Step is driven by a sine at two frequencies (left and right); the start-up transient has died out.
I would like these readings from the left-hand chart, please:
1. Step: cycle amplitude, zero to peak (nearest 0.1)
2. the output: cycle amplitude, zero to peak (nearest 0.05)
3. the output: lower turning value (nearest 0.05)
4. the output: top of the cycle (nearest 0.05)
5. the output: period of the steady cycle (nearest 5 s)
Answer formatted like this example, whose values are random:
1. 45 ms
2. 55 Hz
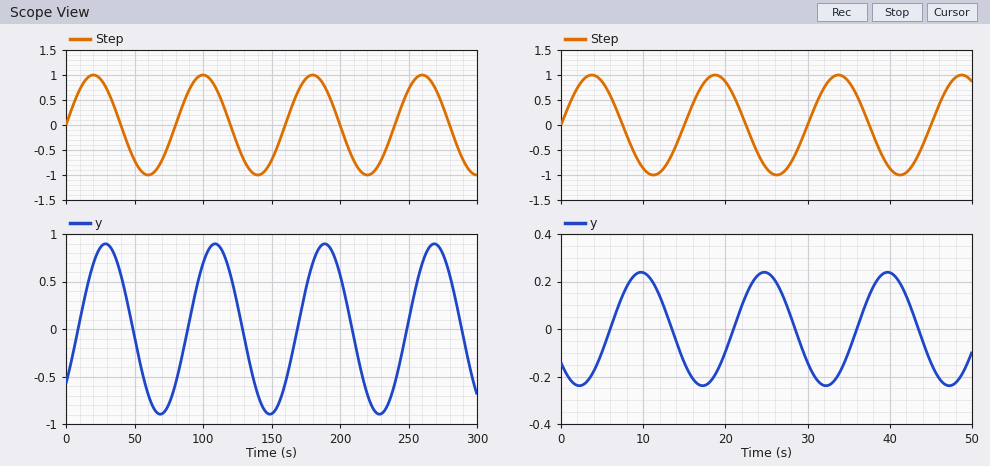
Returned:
1. 1.0
2. 0.90
3. -0.90
4. 0.90
5. 80 s
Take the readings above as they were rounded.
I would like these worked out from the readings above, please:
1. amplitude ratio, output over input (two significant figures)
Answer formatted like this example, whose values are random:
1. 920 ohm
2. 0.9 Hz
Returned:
1. 0.90
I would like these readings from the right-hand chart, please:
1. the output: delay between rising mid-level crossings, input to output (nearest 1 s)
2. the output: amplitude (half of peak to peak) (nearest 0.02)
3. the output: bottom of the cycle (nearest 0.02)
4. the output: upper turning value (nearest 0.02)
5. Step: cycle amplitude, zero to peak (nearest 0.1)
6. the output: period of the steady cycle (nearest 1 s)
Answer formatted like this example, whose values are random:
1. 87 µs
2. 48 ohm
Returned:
1. 6 s
2. 0.24
3. -0.24
4. 0.24
5. 1.0
6. 15 s
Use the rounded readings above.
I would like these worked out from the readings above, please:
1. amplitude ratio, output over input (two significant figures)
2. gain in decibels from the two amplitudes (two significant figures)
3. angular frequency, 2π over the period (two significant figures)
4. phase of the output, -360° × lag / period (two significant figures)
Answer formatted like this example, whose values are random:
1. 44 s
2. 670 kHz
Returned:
1. 0.24
2. -12 dB
3. 0.42 rad/s
4. -140°
